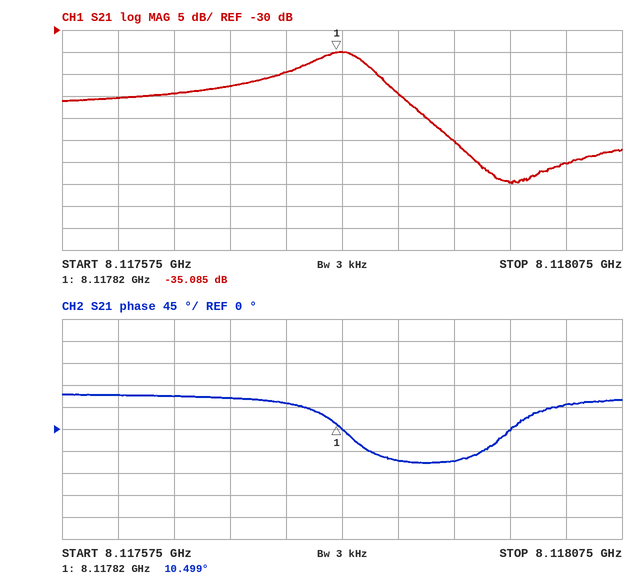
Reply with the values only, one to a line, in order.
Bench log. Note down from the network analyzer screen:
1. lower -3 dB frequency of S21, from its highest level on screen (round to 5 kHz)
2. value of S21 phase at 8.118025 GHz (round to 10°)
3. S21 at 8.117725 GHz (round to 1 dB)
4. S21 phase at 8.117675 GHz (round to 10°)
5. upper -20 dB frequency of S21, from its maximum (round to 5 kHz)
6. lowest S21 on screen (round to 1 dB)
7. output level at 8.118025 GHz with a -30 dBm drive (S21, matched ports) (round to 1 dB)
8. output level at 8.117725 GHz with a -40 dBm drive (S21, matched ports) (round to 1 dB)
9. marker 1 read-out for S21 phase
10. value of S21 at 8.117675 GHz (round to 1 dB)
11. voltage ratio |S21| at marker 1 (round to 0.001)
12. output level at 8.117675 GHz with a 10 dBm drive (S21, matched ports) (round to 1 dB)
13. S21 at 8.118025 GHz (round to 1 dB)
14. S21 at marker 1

8.117790 GHz
50°
-43 dB
70°
8.117925 GHz
-65 dB
-90 dBm
-83 dBm
10.499°
-44 dB
0.018
-34 dBm
-60 dB
-35.085 dB
